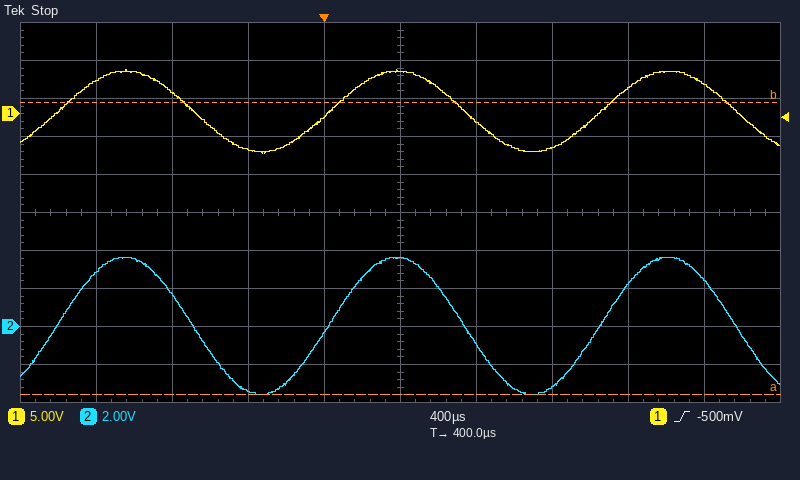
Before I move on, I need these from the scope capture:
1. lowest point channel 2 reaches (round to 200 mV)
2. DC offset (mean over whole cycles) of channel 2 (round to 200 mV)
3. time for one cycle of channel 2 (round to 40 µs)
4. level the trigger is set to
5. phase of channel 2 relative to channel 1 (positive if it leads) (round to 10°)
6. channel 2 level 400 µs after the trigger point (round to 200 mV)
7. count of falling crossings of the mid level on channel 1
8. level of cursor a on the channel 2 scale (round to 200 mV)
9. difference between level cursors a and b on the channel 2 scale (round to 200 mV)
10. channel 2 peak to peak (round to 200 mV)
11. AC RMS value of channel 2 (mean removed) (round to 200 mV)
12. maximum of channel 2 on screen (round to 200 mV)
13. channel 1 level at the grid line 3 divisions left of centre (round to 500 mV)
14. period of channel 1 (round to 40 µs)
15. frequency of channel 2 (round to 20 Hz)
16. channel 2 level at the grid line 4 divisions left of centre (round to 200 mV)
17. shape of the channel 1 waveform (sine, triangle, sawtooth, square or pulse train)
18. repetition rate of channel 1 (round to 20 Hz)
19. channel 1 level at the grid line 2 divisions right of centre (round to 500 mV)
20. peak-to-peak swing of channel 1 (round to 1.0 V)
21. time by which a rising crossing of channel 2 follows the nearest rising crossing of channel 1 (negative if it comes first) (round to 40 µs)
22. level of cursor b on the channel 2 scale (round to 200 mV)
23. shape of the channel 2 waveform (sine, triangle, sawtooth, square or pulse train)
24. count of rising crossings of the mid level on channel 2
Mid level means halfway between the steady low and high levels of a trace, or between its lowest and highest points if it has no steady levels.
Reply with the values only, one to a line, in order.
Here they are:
-3.6 V
0.0 V
1.44 ms
-500 mV
0°
3.6 V
3
-3.6 V
15.4 V
7.2 V
2.6 V
3.6 V
3.0 V
1.44 ms
700 Hz
2.8 V
sine
700 Hz
-4.5 V
11.0 V
0 µs
11.8 V
sine
3
